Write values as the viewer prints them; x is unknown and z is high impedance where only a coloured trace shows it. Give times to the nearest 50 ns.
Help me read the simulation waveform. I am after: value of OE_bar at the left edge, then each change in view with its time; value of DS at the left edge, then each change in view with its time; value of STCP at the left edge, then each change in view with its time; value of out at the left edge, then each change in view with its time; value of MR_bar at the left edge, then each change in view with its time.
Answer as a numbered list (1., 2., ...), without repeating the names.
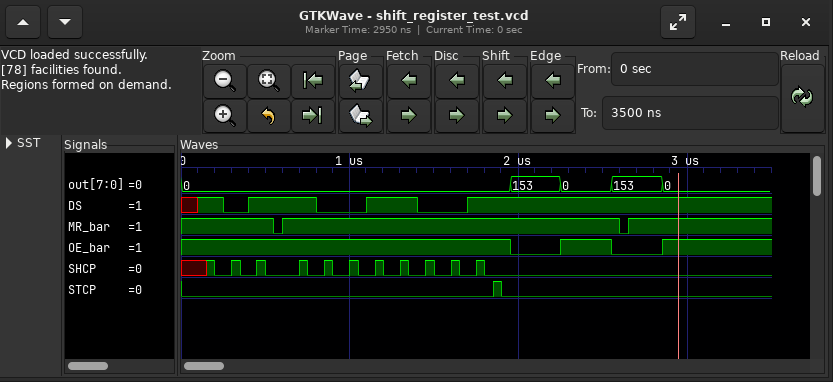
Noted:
1. 1, 0 at 1950 ns, 1 at 2250 ns, 0 at 2550 ns, 1 at 2850 ns
2. x, 1 at 100 ns, 0 at 250 ns, 1 at 400 ns, 0 at 800 ns, 1 at 1100 ns, 0 at 1400 ns, 1 at 1700 ns
3. 0, 1 at 1850 ns, 0 at 1900 ns
4. 0, 153 at 1950 ns, 0 at 2250 ns, 153 at 2550 ns, 0 at 2850 ns
5. 1, 0 at 550 ns, 1 at 600 ns, 0 at 2600 ns, 1 at 2650 ns
